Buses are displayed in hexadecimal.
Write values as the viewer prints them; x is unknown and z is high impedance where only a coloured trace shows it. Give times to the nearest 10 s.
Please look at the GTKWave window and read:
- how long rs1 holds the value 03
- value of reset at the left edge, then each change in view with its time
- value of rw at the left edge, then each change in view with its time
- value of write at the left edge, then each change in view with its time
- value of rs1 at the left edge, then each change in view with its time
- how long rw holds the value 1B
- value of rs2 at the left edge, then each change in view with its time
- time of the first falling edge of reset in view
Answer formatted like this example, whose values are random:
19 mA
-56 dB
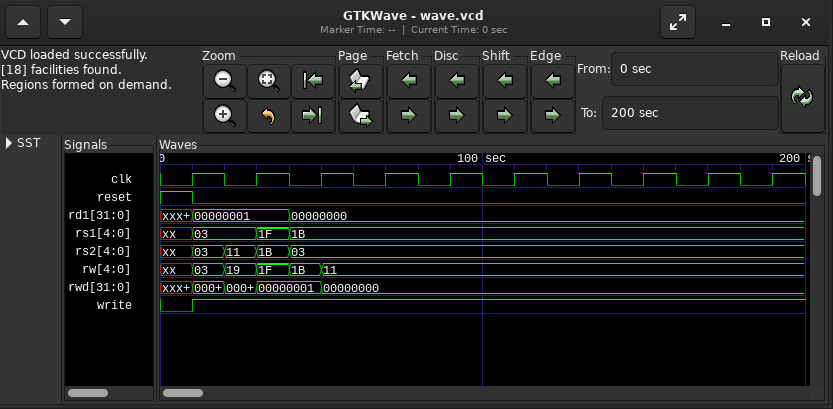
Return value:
20 s
1, 0 at 10 s
xx, 03 at 10 s, 19 at 20 s, 1F at 30 s, 1B at 40 s, 11 at 50 s
0, 1 at 10 s
xx, 03 at 10 s, 1F at 30 s, 1B at 40 s
10 s
xx, 03 at 10 s, 11 at 20 s, 1B at 30 s, 03 at 40 s
10 s
